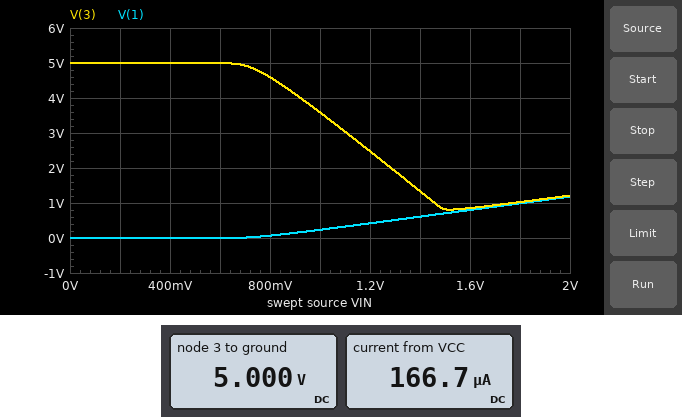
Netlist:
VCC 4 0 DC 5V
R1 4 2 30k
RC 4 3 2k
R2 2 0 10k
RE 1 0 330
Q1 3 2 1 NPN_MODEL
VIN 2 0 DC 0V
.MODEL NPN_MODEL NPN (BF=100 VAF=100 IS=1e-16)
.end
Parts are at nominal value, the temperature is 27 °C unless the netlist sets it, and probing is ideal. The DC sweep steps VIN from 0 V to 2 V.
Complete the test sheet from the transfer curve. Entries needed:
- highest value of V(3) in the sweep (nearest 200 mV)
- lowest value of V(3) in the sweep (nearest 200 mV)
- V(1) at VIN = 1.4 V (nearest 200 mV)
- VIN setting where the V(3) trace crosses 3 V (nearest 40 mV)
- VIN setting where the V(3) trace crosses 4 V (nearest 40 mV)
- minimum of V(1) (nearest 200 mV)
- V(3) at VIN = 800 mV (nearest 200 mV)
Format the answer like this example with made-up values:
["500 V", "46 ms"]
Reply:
["5.0 V", "800 mV", "600 mV", "1.12 V", "920 mV", "0 V", "4.6 V"]
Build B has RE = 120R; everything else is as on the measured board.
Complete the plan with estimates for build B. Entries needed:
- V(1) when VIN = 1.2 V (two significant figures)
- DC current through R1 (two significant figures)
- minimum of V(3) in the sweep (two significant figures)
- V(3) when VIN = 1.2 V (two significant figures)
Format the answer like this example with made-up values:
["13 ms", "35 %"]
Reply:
["390 mV", "170 µA", "370 mV", "430 mV"]
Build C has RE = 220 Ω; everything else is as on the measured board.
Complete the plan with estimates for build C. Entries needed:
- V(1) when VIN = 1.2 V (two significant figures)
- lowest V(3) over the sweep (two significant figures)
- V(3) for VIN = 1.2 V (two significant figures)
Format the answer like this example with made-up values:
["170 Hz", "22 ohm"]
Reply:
["410 mV", "590 mV", "1.3 V"]
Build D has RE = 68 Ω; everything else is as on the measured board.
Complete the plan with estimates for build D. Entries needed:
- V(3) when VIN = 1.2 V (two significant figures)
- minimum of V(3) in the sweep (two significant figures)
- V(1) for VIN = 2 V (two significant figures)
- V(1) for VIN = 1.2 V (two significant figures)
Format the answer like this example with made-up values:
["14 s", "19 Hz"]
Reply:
["400 mV", "240 mV", "1.1 V", "370 mV"]
